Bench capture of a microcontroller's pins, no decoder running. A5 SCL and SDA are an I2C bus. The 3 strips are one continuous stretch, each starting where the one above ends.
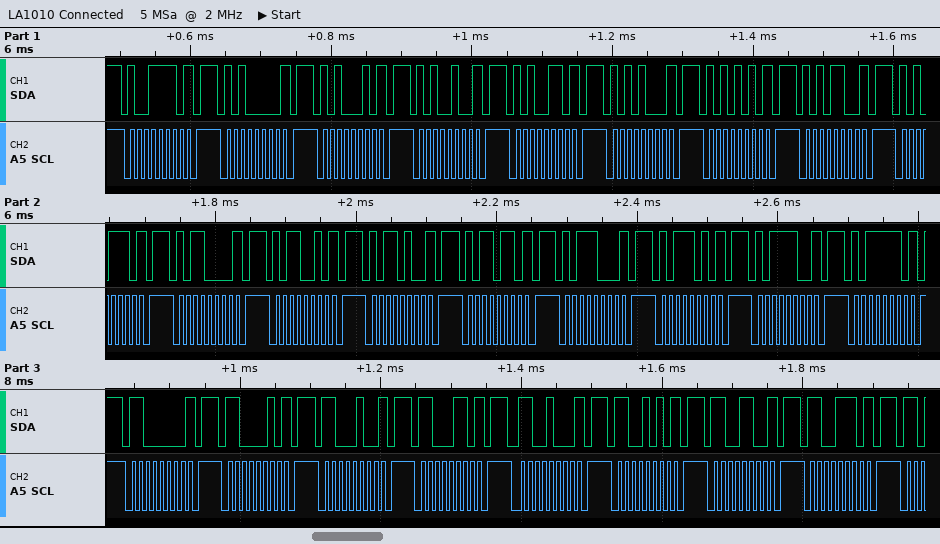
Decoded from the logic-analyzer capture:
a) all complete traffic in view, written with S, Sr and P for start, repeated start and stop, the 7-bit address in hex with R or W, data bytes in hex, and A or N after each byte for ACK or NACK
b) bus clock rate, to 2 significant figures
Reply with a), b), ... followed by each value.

a) S 4FW N P S 50W N P S 51W N P S 52W N P S 53W N P S 54W N P S 55W N P S 56W N P S 57W N P S 58W N P S 59W N P S 5AW N P S 5BW N P S 5CW N P S 5DW N P S 5EW N P S 5FW N P S 60W N P S 61W N P S 62W N P S 63W N P S 64W N P S 65W N P S 66W N P S 67W N P
b) 100 kHz
